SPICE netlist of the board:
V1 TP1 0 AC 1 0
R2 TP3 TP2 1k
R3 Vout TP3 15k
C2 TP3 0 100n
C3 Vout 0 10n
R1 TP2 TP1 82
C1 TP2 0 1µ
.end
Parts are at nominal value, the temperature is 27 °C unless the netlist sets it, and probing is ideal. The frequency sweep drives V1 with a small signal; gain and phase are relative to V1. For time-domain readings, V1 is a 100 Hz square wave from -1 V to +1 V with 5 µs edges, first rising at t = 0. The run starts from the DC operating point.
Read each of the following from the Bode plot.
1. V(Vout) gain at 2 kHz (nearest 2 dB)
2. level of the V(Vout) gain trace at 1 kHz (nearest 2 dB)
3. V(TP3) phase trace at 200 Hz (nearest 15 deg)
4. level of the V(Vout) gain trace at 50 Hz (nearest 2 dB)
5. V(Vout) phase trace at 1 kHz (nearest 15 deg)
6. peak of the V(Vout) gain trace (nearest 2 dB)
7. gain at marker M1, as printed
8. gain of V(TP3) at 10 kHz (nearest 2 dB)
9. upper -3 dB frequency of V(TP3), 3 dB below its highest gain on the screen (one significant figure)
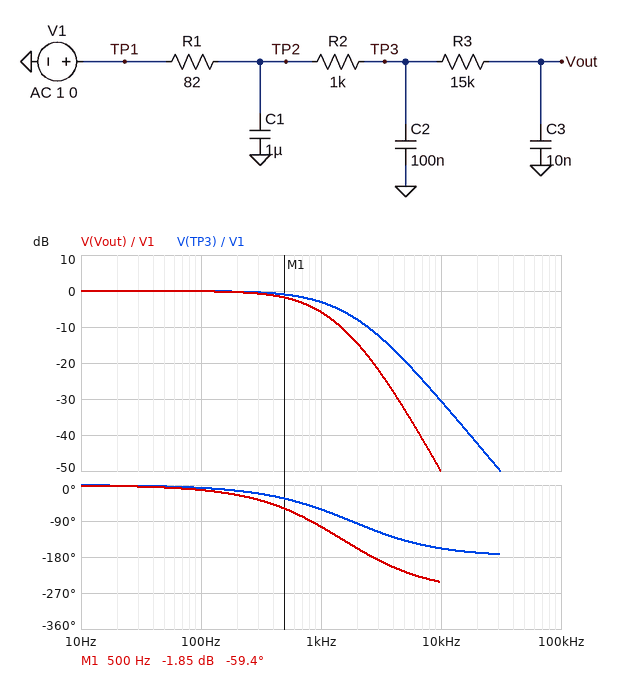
-14 dB
-6 dB
-15 deg
0 dB
-105 deg
0 dB
-1.85 dB
-30 dB
1 kHz
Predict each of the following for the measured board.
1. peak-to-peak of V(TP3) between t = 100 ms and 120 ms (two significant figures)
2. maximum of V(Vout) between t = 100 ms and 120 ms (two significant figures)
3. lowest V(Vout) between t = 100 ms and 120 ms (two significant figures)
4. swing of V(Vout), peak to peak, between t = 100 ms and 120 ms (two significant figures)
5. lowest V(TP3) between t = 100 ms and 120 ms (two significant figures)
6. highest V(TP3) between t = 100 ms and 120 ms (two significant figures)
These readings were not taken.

2.0 V
1.0 V
-1.0 V
2.0 V
-1.0 V
1.0 V
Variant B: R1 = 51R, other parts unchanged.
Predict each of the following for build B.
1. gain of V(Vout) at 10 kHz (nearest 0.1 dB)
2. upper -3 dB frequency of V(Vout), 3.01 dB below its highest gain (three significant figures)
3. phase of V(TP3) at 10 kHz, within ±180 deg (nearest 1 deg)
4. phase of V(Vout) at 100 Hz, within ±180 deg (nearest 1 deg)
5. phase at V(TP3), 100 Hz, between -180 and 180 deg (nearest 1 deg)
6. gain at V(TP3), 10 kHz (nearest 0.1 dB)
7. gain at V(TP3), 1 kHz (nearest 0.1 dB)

-46.2 dB
714 Hz
-152 deg
-11 deg
-6 deg
-26.7 dB
-2.4 dB
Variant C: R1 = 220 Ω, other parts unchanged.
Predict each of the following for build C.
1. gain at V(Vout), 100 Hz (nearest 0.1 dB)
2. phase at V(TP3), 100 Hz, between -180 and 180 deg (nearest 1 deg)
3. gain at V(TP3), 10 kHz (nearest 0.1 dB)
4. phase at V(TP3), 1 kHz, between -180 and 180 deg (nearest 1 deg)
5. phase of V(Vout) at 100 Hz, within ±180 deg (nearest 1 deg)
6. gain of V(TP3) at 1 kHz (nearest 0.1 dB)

-0.2 dB
-13 deg
-39.0 dB
-87 deg
-18 deg
-7.0 dB
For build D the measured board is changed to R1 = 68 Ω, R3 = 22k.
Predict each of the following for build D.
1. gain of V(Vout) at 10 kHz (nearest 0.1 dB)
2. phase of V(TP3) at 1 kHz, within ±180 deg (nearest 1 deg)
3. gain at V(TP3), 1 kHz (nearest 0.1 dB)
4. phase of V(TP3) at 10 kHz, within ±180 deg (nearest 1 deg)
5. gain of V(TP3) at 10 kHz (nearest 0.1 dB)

-51.8 dB
-56 deg
-2.7 dB
-157 deg
-29.0 dB
